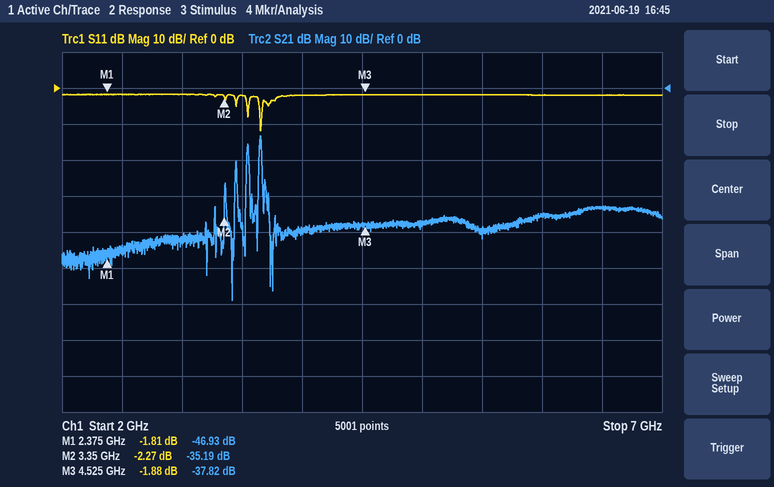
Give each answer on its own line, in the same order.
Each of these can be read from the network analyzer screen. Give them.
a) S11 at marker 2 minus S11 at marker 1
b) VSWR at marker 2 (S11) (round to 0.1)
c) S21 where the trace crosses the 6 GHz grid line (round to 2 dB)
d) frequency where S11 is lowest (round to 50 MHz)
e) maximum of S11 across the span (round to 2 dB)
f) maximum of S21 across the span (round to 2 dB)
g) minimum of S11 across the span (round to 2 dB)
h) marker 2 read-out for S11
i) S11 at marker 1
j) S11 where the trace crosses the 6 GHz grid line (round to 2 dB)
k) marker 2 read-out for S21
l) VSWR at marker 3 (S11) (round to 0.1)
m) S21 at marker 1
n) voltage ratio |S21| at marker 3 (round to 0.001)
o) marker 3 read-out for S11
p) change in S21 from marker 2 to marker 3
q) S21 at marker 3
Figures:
-0.46 dB
7.7
-36 dB
3.65 GHz
-2 dB
-14 dB
-12 dB
-2.27 dB
-1.81 dB
-2 dB
-35.19 dB
9.3
-46.93 dB
0.013
-1.88 dB
-2.63 dB
-37.82 dB
